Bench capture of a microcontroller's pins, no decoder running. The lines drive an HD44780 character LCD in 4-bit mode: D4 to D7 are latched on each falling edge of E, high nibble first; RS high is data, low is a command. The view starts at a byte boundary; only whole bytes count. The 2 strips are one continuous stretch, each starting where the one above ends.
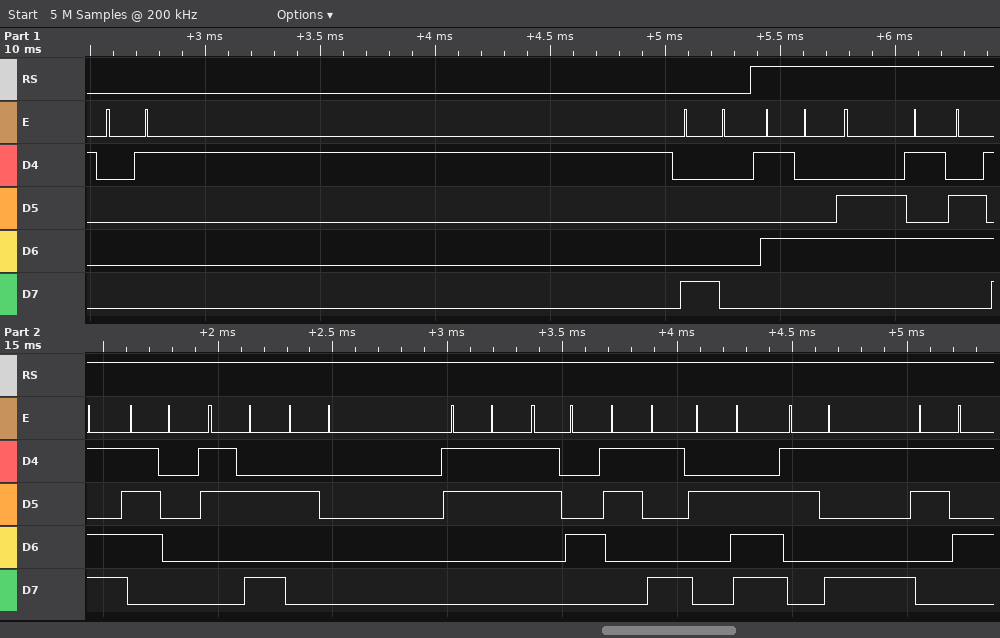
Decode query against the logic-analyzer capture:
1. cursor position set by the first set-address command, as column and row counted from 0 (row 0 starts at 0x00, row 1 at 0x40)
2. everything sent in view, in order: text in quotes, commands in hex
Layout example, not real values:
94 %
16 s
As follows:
column 0, row 0
0x01 0x80 "Temp: 349.95"
